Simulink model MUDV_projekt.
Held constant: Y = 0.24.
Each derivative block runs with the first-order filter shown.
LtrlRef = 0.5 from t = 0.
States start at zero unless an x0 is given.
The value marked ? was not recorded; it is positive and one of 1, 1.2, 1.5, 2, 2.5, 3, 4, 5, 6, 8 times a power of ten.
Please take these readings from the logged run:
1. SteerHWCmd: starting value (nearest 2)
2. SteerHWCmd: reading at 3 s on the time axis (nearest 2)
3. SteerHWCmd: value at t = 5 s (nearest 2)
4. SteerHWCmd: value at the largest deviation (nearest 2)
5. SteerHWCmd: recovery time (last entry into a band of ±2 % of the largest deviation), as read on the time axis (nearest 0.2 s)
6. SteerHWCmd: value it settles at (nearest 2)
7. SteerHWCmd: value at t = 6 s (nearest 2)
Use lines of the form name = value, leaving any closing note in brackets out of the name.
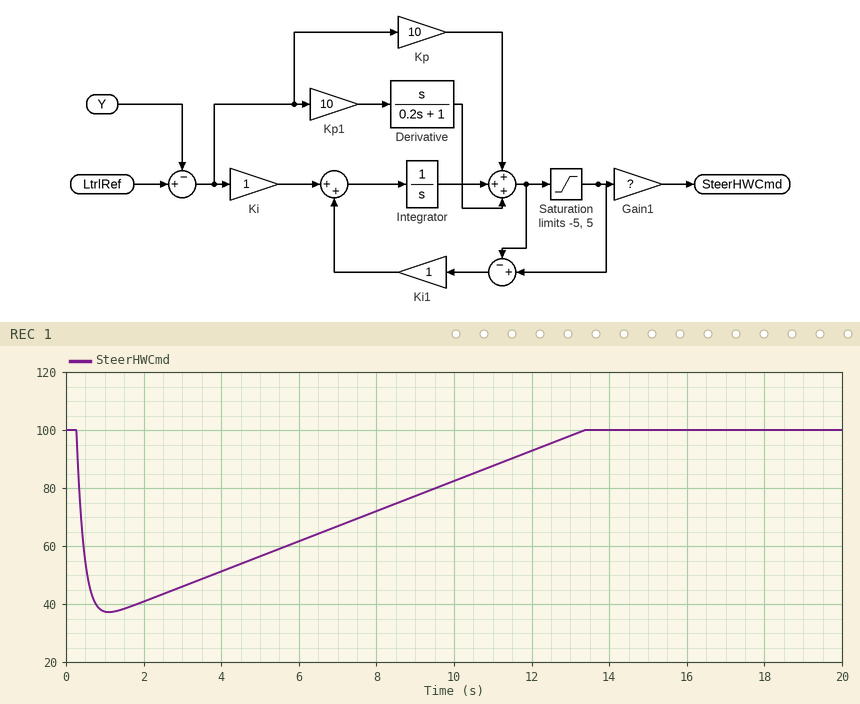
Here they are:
SteerHWCmd: starting value = 100
SteerHWCmd: reading at 3 s on the time axis = 46
SteerHWCmd: value at t = 5 s = 56
SteerHWCmd: value at the largest deviation = 38
SteerHWCmd: recovery time (last entry into a band of ±2 % of the largest deviation), as read on the time axis = 13.2 s
SteerHWCmd: value it settles at = 100
SteerHWCmd: value at t = 6 s = 62
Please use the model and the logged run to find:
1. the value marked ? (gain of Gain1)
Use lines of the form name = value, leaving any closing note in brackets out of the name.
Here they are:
the value marked ? = 20
